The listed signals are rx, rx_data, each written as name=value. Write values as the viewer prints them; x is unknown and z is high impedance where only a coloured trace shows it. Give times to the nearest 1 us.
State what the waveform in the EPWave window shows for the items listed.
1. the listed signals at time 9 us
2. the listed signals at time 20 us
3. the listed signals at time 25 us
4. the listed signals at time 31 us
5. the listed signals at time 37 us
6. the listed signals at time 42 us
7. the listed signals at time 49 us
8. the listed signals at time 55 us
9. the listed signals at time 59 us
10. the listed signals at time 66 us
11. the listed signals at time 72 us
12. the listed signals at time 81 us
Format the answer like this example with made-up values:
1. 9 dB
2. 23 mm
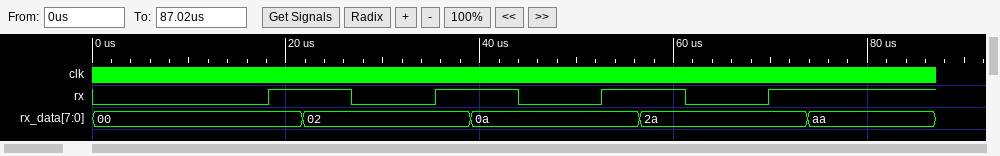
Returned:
1. rx=0, rx_data=00
2. rx=1, rx_data=00
3. rx=1, rx_data=02
4. rx=0, rx_data=02
5. rx=1, rx_data=02
6. rx=1, rx_data=0a
7. rx=0, rx_data=0a
8. rx=1, rx_data=0a
9. rx=1, rx_data=2a
10. rx=0, rx_data=2a
11. rx=1, rx_data=2a
12. rx=1, rx_data=aa
